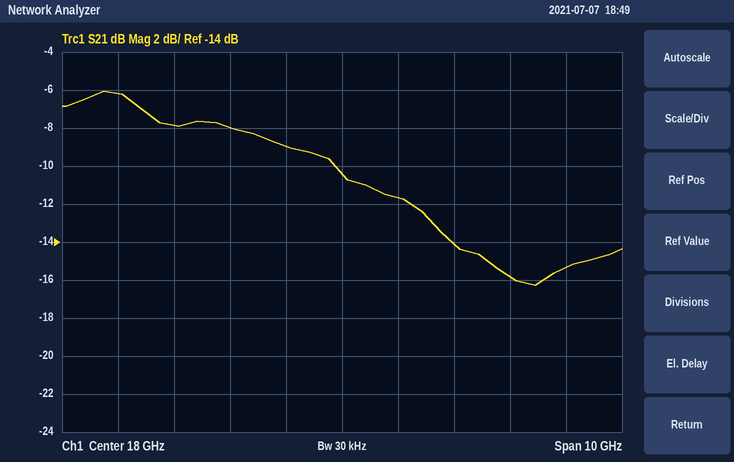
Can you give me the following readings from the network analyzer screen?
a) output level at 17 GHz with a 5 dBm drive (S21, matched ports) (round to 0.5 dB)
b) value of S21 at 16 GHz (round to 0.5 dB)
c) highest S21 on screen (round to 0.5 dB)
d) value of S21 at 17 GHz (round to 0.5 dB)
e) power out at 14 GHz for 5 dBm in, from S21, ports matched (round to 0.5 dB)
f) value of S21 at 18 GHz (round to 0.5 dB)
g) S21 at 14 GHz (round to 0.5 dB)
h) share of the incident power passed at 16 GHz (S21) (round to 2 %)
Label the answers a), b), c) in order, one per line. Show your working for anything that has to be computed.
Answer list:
a) 5 dBm + (-9.0 dB) = -4.0 dBm
b) -8.0 dB
c) -6.0 dB
d) -9.0 dB
e) 5 dBm + (-6.0 dB) = -1.0 dBm
f) -10.5 dB
g) -6.0 dB
h) 10^(-8/10) ≈ 16 %
